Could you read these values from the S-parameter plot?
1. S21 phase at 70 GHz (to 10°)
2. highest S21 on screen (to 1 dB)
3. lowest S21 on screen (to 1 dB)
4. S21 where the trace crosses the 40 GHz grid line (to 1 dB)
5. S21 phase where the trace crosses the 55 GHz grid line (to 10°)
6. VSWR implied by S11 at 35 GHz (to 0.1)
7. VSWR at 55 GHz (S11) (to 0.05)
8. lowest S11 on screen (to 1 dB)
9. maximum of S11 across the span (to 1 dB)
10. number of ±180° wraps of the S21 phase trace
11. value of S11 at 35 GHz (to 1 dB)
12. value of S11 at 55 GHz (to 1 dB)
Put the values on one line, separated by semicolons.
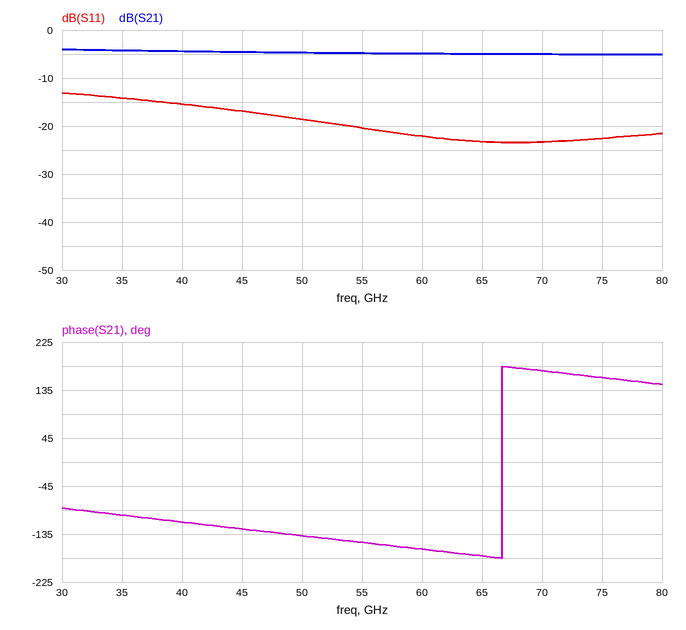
170°; -4 dB; -5 dB; -4 dB; -150°; 1.5; 1.20; -23 dB; -13 dB; 1; -14 dB; -20 dB
